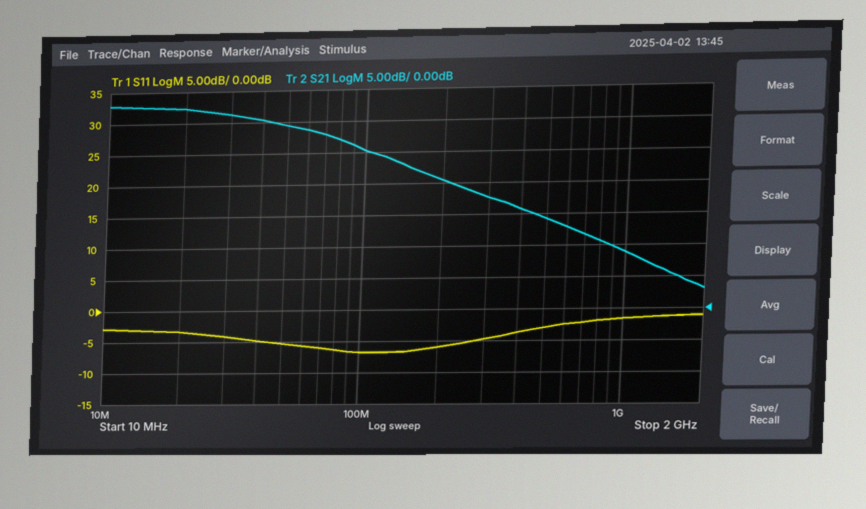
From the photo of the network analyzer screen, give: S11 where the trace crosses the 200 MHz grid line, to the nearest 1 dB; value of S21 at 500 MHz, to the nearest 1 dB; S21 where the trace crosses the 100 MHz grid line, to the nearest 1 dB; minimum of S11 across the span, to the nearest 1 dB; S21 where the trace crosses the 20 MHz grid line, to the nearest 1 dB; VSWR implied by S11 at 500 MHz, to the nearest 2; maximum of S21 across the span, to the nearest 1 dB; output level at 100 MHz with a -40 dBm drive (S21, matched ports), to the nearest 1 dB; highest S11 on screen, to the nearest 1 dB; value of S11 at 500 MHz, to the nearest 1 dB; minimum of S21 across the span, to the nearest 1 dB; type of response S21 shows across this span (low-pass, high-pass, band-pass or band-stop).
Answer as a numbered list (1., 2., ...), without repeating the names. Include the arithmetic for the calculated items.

1. -6 dB
2. 14 dB
3. 25 dB
4. -7 dB
5. 32 dB
6. |Γ| = 10^(-3/20) = 0.7079; VSWR = (1 + 0.7079)/(1 − 0.7079) ≈ 6
7. 33 dB
8. -40 dBm + (25 dB) = -15 dBm
9. -1 dB
10. -3 dB
11. 3 dB
12. low-pass
